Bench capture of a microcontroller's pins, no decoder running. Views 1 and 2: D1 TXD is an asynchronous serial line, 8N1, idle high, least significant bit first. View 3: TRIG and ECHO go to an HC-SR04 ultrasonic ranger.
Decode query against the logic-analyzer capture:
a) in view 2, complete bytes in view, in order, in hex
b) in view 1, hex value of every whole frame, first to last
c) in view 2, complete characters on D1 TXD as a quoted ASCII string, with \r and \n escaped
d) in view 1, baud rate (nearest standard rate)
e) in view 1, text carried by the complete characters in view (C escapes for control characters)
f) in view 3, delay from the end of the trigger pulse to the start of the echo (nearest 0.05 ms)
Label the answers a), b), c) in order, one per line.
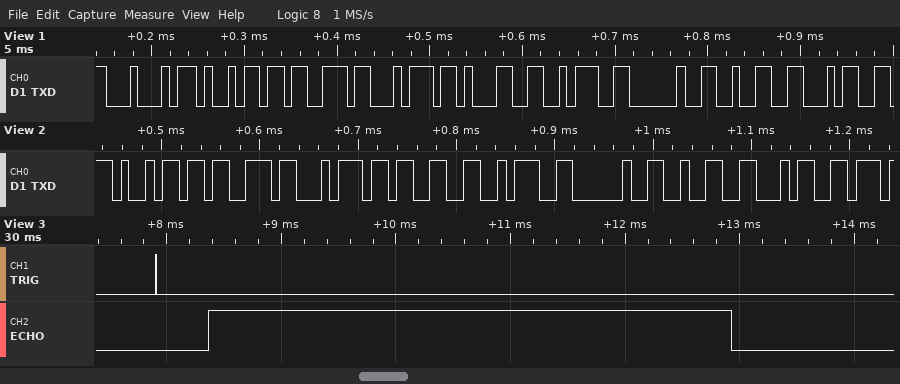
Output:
a) 0x69 0x73 0x74 0x33 0x3A 0x20 0x32 0x34
b) 44 69 73 74 31 3A 20 32 34
c) "ist3: 24"
d) 115200 baud
e) "Dist1: 24"
f) 0.45 ms
